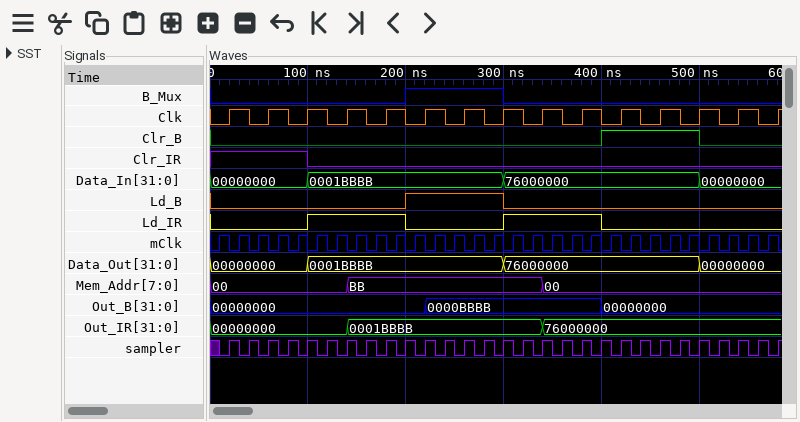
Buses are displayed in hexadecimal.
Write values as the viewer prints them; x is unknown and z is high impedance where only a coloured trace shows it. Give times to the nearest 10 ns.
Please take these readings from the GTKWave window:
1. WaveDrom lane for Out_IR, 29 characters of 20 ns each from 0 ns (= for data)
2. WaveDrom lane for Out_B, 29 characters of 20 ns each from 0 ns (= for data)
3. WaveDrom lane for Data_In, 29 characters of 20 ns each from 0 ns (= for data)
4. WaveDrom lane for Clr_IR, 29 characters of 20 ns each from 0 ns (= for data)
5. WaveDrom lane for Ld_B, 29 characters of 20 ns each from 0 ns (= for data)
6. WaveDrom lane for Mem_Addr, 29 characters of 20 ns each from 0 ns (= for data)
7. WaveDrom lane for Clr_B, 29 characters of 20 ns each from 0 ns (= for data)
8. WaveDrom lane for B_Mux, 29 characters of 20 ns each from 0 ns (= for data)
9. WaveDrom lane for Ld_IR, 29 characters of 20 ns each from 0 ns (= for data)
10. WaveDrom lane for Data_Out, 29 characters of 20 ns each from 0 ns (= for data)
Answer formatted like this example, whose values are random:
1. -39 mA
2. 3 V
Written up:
1. {name: 'Out_IR', wave: '=......=.........=...........', data: '00000000 0001BBBB 76000000'}
2. {name: 'Out_B', wave: '=..........=........=........', data: '00000000 0000BBBB 00000000'}
3. {name: 'Data_In', wave: '=....=.........=.........=...', data: '00000000 0001BBBB 76000000 00000000'}
4. {name: 'Clr_IR', wave: '1....0.......................'}
5. {name: 'Ld_B', wave: '0.........1....0.............'}
6. {name: 'Mem_Addr', wave: '=......=.........=...........', data: '00 BB 00'}
7. {name: 'Clr_B', wave: '0...................1....0...'}
8. {name: 'B_Mux', wave: '0.........1....0.............'}
9. {name: 'Ld_IR', wave: '0....1....0....1....0........'}
10. {name: 'Data_Out', wave: '=....=.........=.........=...', data: '00000000 0001BBBB 76000000 00000000'}
